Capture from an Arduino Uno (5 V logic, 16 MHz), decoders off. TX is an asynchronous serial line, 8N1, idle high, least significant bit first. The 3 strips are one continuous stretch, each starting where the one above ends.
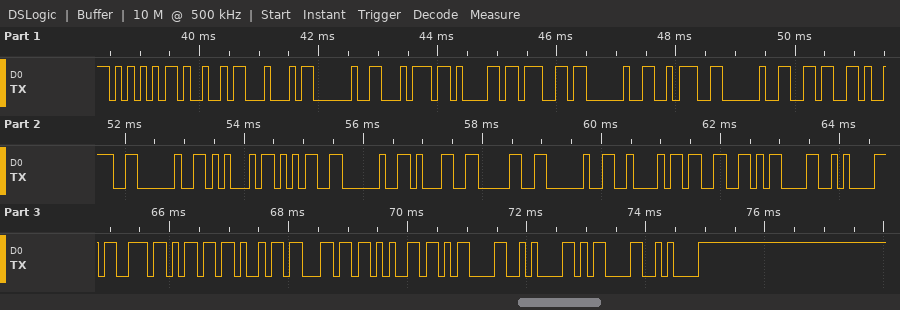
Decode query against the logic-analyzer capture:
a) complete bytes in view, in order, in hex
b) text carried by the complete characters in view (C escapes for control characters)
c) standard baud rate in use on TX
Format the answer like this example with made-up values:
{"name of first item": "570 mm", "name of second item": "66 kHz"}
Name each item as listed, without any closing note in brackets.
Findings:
{"complete bytes in view, in order, in hex": "55 49 44 20 74 61 67 20 3A 20 36 39 20 45 35 20 31 30 20 42 33 0D 0A 73 6D 69 6C 65 0D 0A 0D 0A", "text carried by the complete characters in view": "\"UID tag : 69 E5 10 B3\\r\\nsmile\\r\\n\\r\\n\"", "standard baud rate in use on TX": "9600 baud"}
